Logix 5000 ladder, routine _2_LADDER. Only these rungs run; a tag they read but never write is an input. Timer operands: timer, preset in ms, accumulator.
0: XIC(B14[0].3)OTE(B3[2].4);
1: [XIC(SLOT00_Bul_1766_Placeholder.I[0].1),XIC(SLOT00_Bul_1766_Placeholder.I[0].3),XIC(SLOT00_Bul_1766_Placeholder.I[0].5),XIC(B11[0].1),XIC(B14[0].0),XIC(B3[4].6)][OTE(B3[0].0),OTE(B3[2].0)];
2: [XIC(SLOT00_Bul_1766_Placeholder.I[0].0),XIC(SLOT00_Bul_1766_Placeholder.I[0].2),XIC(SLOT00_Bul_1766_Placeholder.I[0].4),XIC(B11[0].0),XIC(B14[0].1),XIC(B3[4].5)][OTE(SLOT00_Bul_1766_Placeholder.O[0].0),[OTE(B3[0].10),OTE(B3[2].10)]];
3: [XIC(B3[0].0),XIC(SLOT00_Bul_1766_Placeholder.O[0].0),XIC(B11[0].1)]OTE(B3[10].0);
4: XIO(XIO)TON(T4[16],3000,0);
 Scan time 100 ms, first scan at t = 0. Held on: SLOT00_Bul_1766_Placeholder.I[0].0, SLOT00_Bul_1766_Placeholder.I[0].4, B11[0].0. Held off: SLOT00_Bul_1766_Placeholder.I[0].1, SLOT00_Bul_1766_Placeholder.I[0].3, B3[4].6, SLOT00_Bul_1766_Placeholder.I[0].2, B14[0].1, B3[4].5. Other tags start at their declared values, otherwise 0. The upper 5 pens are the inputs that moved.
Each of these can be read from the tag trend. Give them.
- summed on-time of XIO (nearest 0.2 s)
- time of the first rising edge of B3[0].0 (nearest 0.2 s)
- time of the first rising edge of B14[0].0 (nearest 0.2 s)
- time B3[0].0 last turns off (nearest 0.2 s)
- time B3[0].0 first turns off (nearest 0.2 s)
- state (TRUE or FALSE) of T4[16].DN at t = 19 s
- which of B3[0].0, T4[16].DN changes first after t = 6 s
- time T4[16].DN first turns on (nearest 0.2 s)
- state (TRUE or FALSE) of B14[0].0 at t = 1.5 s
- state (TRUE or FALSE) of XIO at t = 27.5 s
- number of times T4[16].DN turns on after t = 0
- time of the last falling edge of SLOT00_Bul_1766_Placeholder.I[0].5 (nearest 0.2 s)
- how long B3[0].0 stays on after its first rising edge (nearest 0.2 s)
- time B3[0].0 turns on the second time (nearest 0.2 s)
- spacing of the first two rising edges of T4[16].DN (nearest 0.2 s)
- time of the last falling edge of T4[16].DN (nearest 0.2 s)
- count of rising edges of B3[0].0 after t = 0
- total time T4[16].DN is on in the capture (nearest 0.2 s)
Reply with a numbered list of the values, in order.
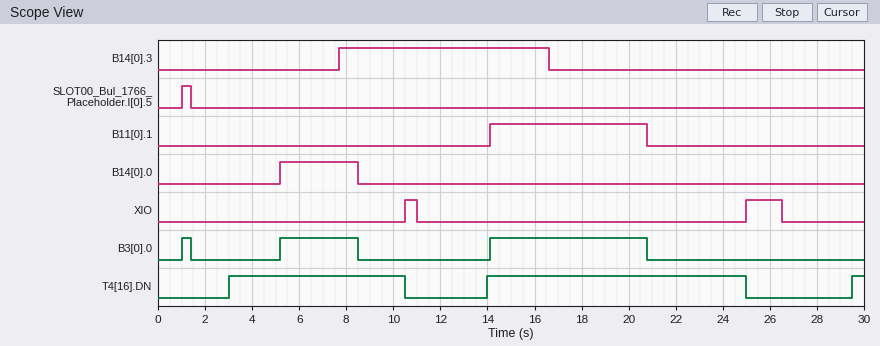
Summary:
1. 2.0 s
2. 1.0 s
3. 5.2 s
4. 20.8 s
5. 1.4 s
6. TRUE
7. B3[0].0
8. 3.0 s
9. FALSE
10. FALSE
11. 3
12. 1.4 s
13. 0.4 s
14. 5.2 s
15. 11.0 s
16. 25.0 s
17. 3
18. 19.0 s
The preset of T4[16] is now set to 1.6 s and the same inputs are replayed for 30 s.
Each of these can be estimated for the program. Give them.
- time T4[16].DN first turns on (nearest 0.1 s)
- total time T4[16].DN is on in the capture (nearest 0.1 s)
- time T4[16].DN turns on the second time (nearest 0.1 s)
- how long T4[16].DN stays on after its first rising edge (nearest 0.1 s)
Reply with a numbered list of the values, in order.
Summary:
1. 1.6 s
2. 23.2 s
3. 12.6 s
4. 8.9 s
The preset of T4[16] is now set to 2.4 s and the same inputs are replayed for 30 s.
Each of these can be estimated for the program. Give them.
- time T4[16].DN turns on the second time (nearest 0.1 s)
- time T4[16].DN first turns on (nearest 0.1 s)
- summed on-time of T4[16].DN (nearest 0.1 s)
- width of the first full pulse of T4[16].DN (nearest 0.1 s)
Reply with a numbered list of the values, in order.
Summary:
1. 13.4 s
2. 2.4 s
3. 20.8 s
4. 8.1 s
